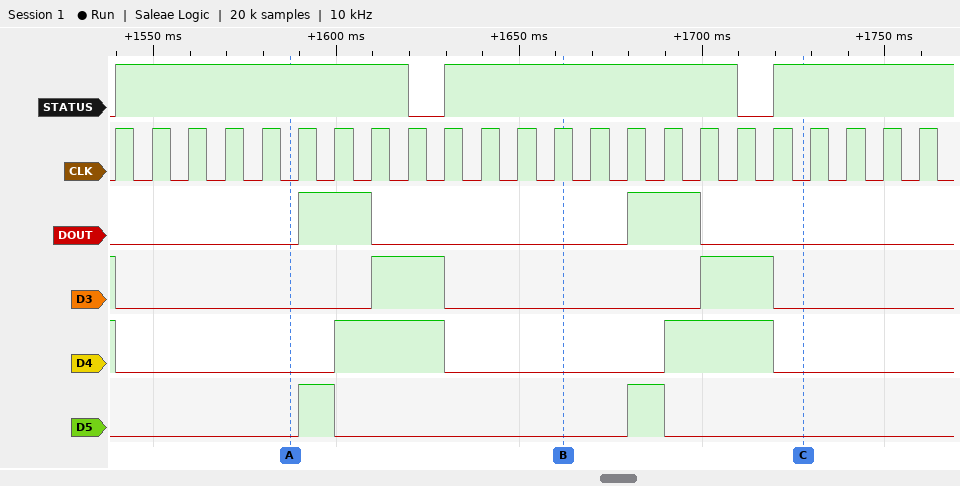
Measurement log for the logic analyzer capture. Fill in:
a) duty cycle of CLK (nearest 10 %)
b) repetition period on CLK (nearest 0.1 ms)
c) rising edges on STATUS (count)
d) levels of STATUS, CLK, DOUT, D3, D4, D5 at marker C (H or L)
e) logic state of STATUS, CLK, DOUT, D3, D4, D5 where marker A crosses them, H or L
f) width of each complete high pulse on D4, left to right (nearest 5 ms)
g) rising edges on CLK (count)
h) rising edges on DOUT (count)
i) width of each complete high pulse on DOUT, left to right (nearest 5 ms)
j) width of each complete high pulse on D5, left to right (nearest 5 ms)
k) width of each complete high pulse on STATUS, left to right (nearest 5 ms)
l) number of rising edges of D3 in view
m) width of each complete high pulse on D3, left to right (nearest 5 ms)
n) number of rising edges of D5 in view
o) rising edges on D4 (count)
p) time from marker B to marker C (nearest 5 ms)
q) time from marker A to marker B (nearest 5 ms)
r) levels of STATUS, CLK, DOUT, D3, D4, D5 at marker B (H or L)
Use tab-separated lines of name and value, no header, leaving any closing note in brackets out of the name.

duty cycle of CLK	50 %
repetition period on CLK	10 ms
rising edges on STATUS	3
levels of STATUS, CLK, DOUT, D3, D4, D5 at marker C	STATUS=H, CLK=L, DOUT=L, D3=L, D4=L, D5=L
logic state of STATUS, CLK, DOUT, D3, D4, D5 where marker A crosses them, H or L	STATUS=H, CLK=L, DOUT=L, D3=L, D4=L, D5=L
width of each complete high pulse on D4, left to right	30 ms, 30 ms
rising edges on CLK	23
rising edges on DOUT	2
width of each complete high pulse on DOUT, left to right	20 ms, 20 ms
width of each complete high pulse on D5, left to right	10 ms, 10 ms
width of each complete high pulse on STATUS, left to right	80 ms, 80 ms
number of rising edges of D3 in view	2
width of each complete high pulse on D3, left to right	20 ms, 20 ms
number of rising edges of D5 in view	2
rising edges on D4	2
time from marker B to marker C	65 ms
time from marker A to marker B	75 ms
levels of STATUS, CLK, DOUT, D3, D4, D5 at marker B	STATUS=H, CLK=H, DOUT=L, D3=L, D4=L, D5=L
